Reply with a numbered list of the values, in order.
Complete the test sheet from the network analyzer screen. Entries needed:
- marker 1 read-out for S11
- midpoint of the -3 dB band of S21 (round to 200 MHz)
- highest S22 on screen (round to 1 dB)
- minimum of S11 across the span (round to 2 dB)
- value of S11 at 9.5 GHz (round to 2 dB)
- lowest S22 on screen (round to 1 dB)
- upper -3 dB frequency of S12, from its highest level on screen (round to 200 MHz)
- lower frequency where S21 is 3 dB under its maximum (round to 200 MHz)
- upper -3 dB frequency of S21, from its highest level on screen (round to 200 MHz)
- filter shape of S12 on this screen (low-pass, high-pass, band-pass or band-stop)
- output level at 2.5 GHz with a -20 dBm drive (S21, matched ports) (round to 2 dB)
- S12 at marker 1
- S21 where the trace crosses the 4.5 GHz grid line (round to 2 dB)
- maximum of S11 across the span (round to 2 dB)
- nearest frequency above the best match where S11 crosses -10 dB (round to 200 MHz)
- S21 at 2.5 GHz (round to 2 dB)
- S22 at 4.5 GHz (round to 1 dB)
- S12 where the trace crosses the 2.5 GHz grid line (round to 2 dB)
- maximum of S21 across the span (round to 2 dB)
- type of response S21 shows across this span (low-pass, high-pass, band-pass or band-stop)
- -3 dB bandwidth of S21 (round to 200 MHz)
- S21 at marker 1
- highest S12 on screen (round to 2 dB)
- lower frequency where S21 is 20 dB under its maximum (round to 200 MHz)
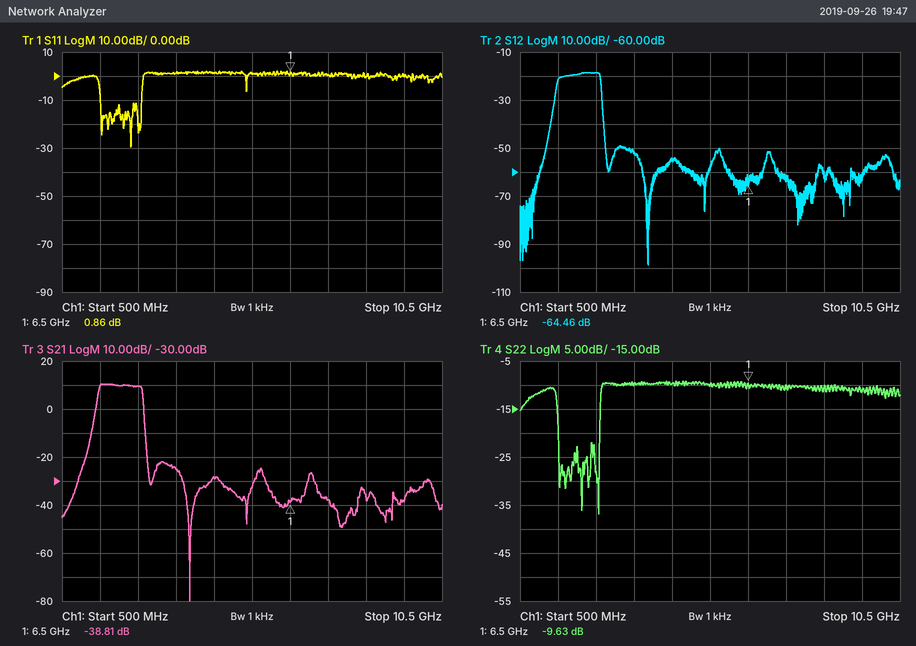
1. 0.86 dB
2. 2.0 GHz
3. -9 dB
4. -30 dB
5. 0 dB
6. -37 dB
7. 2.6 GHz
8. 1.4 GHz
9. 2.6 GHz
10. band-pass
11. -10 dBm
12. -64.46 dB
13. -28 dB
14. 2 dB
15. 2.6 GHz
16. 10 dB
17. -10 dB
18. -18 dB
19. 10 dB
20. band-pass
21. 1.2 GHz
22. -38.81 dB
23. -18 dB
24. 1.2 GHz
